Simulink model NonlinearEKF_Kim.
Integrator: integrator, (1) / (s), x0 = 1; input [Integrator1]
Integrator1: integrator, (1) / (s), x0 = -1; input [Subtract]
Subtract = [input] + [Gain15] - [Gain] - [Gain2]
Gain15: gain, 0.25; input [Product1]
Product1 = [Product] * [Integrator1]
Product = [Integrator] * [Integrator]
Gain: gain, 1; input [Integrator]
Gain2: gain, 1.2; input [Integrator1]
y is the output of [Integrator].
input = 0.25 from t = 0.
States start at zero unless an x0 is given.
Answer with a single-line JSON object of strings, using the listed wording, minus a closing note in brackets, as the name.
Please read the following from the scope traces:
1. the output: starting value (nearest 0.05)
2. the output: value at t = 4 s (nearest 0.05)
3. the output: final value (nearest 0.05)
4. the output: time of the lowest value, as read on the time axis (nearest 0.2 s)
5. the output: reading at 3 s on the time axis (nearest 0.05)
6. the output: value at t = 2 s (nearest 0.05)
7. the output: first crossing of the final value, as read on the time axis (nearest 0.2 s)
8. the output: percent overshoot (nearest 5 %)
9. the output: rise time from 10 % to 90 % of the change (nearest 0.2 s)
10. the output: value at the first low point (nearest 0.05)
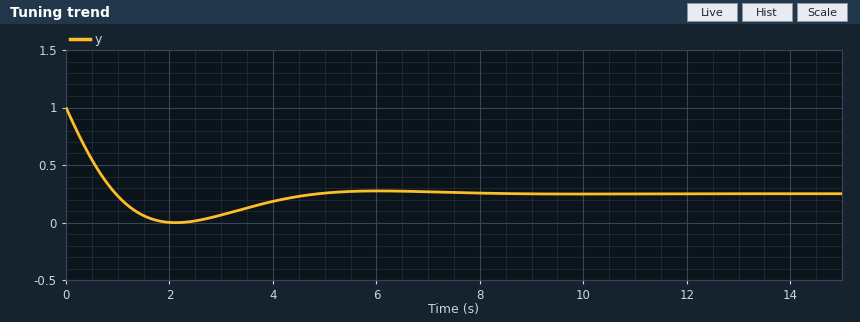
{"the output: starting value": "1.00", "the output: value at t = 4 s": "0.20", "the output: final value": "0.25", "the output: time of the lowest value, as read on the time axis": "2.2 s", "the output: reading at 3 s on the time axis": "0.05", "the output: value at t = 2 s": "0.00", "the output: first crossing of the final value, as read on the time axis": "1.0 s", "the output: percent overshoot": "35 %", "the output: rise time from 10 % to 90 % of the change": "0.8 s", "the output: value at the first low point": "0.00"}
